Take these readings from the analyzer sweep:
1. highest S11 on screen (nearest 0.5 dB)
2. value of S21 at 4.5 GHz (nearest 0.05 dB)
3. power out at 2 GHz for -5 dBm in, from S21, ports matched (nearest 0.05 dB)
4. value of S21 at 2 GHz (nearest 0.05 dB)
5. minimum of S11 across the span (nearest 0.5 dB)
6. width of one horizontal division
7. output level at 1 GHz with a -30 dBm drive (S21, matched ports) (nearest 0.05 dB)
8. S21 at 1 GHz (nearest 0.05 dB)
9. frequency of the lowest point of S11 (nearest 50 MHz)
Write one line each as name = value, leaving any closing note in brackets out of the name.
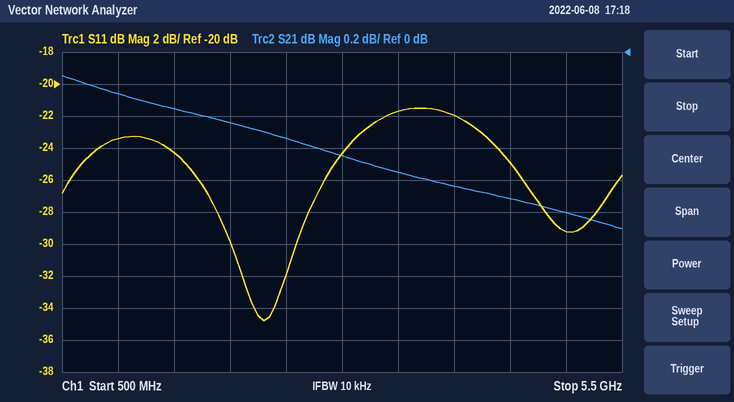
highest S11 on screen = -21.5 dB
value of S21 at 4.5 GHz = -0.90 dB
power out at 2 GHz for -5 dBm in, from S21, ports matched = -5.45 dBm
value of S21 at 2 GHz = -0.45 dB
minimum of S11 across the span = -35.0 dB
width of one horizontal division = 500 MHz
output level at 1 GHz with a -30 dBm drive (S21, matched ports) = -30.25 dBm
S21 at 1 GHz = -0.25 dB
frequency of the lowest point of S11 = 2.30 GHz
